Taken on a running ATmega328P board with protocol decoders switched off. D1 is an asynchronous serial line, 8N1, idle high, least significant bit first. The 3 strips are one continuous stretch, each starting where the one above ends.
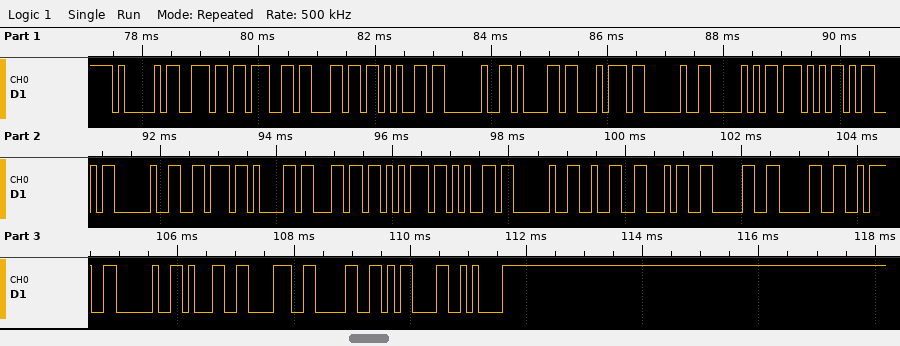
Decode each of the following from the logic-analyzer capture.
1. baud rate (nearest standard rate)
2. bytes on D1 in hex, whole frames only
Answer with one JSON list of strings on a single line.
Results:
["9600 baud", "0x41 0x6E 0x67 0x6C 0x65 0x20 0x61 0x74 0x20 0x50 0x57 0x4D 0x20 0x76 0x61 0x6C 0x75 0x65 0x20 0x32 0x34 0x30 0x30 0x3A 0x20 0x31 0x38 0x30 0x0D 0x0A"]
